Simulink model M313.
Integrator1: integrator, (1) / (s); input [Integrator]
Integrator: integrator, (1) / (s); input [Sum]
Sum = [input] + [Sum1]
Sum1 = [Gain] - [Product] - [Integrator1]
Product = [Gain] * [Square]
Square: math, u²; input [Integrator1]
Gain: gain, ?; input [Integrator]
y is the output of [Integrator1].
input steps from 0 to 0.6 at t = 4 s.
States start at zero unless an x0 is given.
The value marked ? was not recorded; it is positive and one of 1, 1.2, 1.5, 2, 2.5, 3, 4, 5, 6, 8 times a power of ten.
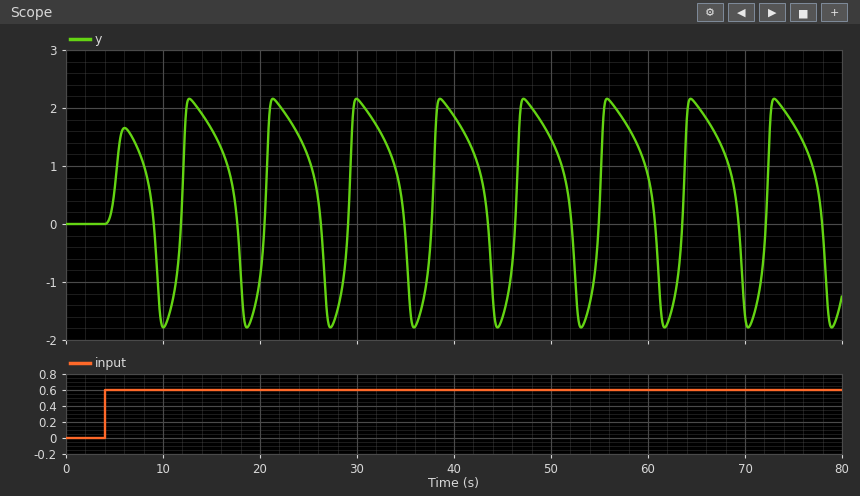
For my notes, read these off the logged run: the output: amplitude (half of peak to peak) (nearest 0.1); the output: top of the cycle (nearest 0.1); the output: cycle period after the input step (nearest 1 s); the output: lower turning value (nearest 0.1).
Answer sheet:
2.0
2.2
9 s
-1.8
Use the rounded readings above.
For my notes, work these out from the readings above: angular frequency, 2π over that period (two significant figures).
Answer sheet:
0.70 rad/s
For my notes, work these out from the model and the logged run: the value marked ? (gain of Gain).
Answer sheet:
2
